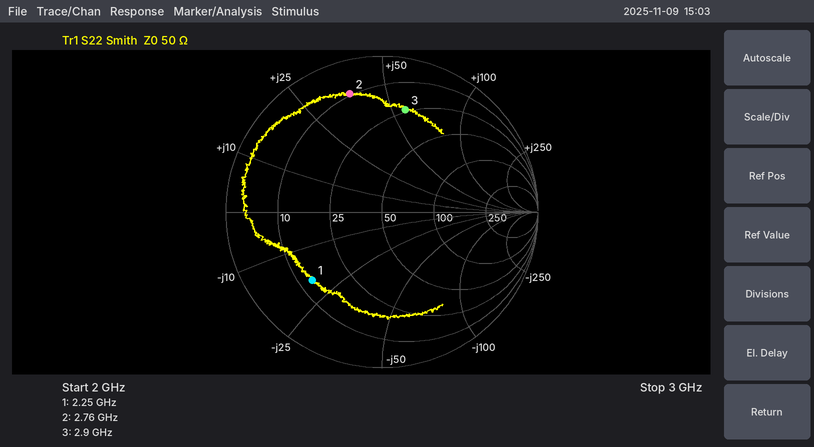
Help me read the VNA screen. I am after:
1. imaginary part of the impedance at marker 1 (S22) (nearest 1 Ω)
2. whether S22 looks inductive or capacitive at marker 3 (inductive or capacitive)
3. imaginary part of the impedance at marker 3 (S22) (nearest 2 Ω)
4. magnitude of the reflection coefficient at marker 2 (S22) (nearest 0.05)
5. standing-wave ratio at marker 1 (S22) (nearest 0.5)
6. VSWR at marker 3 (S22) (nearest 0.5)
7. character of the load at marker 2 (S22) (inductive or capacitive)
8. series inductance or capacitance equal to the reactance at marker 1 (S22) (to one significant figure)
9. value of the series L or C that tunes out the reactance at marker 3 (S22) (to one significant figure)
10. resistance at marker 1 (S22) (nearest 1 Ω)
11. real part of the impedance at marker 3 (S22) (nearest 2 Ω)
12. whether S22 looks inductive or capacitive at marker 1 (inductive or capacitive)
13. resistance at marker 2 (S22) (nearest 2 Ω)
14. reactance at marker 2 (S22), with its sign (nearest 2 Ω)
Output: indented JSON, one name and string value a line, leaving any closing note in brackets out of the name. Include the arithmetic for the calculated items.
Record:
{
  "imaginary part of the impedance at marker 1 (S22)": "-19 Ω",
  "whether S22 looks inductive or capacitive at marker 3": "inductive",
  "imaginary part of the impedance at marker 3 (S22)": "+56 Ω",
  "magnitude of the reflection coefficient at marker 2 (S22)": "0.80",
  "standing-wave ratio at marker 1 (S22)": "4.5",
  "VSWR at marker 3 (S22)": "5.0",
  "character of the load at marker 2 (S22)": "inductive",
  "series inductance or capacitance equal to the reactance at marker 1 (S22)": "C = 1/(2π × 2.25 GHz × 19 Ω) ≈ 4 pF",
  "value of the series L or C that tunes out the reactance at marker 3 (S22)": "C = 1/(2π × 2.9 GHz × 56 Ω) ≈ 1.0 pF",
  "resistance at marker 1 (S22)": "13 Ω",
  "real part of the impedance at marker 3 (S22)": "24 Ω",
  "whether S22 looks inductive or capacitive at marker 1": "capacitive",
  "resistance at marker 2 (S22)": "10 Ω",
  "reactance at marker 2 (S22), with its sign": "+38 Ω"
}
